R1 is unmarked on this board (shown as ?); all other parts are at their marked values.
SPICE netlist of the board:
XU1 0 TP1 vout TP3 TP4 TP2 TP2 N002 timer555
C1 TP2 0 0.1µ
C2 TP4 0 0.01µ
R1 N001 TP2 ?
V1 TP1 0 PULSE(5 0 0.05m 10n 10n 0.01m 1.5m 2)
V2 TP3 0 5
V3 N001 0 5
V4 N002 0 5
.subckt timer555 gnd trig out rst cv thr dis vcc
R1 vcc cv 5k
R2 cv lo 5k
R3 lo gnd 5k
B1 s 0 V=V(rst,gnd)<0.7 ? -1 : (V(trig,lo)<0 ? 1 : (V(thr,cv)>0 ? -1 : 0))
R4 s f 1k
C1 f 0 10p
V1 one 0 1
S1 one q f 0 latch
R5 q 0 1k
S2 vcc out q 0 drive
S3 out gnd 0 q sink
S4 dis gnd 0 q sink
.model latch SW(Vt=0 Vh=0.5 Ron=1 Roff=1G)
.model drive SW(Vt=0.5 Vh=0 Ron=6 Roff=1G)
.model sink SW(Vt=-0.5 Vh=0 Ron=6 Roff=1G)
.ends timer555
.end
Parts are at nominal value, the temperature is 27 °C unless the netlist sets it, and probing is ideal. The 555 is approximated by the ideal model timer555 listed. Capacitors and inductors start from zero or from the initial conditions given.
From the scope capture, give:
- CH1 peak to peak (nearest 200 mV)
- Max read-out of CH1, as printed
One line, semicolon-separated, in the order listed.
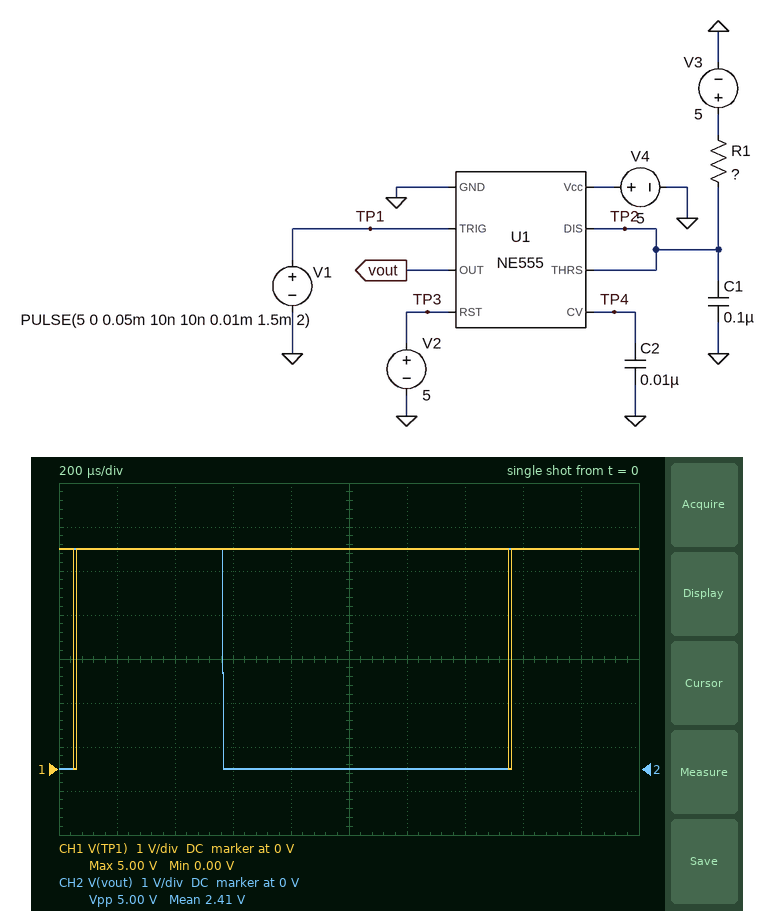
5.0 V; 5.00 V
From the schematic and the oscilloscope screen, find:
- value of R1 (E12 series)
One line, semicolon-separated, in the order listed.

4.7 kΩ
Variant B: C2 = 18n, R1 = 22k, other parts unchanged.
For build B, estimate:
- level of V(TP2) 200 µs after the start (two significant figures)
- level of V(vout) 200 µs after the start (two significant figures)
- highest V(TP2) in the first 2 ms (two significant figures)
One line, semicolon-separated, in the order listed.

330 mV; 5.0 V; 2.9 V
